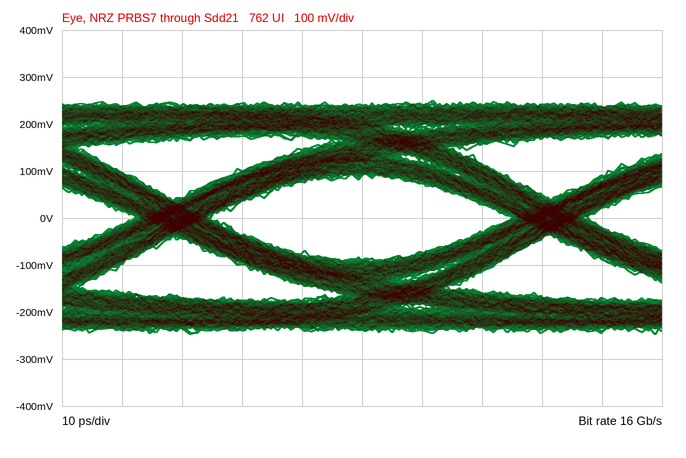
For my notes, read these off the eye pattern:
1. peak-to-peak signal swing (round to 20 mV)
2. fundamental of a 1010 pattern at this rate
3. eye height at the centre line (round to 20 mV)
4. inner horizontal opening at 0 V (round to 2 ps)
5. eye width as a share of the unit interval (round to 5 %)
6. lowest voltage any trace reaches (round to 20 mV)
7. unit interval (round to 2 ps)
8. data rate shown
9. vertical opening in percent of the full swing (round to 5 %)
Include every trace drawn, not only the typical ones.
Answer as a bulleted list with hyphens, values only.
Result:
- 500 mV
- 8 GHz
- 180 mV
- 50 ps
- 80 %
- -240 mV
- 62 ps
- 16 Gb/s
- 35 %
